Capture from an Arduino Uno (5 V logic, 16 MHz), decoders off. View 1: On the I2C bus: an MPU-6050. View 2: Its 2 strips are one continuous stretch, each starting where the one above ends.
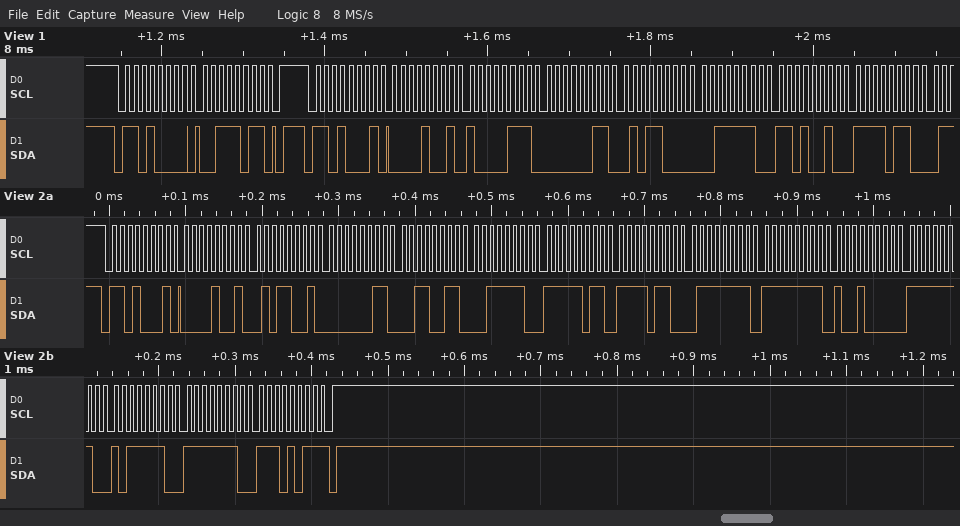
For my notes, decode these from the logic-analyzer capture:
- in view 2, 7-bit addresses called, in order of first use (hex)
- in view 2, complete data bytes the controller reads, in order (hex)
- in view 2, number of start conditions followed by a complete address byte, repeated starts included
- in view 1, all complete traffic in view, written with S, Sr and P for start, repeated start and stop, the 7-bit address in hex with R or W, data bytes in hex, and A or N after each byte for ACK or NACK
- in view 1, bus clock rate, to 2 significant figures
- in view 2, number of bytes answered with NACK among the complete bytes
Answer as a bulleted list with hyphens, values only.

- 0x68
- 09 59 03 33 3E FB F6 7F FF 90 FE BE FE EB
- 1
- S 68W A 3B A P S 68R A 09 A 87 A 03 A 58 A 3E A D2 A F6 A
- 100 kHz
- 1
